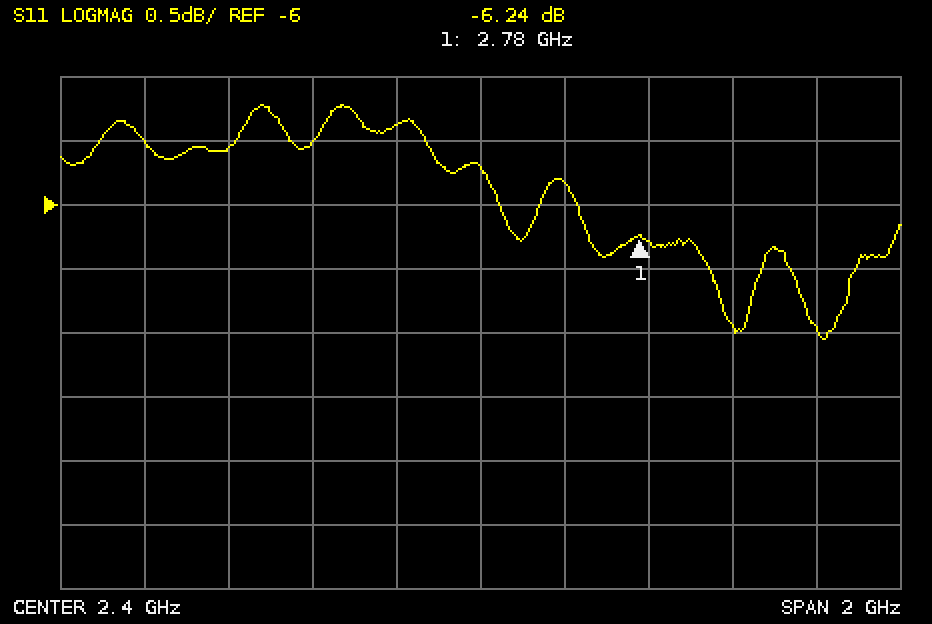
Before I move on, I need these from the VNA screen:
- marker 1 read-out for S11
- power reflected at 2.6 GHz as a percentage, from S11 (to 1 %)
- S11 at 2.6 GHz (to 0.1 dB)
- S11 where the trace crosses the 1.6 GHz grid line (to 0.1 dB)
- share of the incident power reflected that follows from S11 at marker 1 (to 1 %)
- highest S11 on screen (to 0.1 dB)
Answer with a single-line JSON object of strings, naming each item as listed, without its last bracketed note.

{"marker 1 read-out for S11": "-6.24 dB", "power reflected at 2.6 GHz as a percentage, from S11": "26 %", "S11 at 2.6 GHz": "-5.8 dB", "S11 where the trace crosses the 1.6 GHz grid line": "-5.5 dB", "share of the incident power reflected that follows from S11 at marker 1": "24 %", "highest S11 on screen": "-5.2 dB"}
